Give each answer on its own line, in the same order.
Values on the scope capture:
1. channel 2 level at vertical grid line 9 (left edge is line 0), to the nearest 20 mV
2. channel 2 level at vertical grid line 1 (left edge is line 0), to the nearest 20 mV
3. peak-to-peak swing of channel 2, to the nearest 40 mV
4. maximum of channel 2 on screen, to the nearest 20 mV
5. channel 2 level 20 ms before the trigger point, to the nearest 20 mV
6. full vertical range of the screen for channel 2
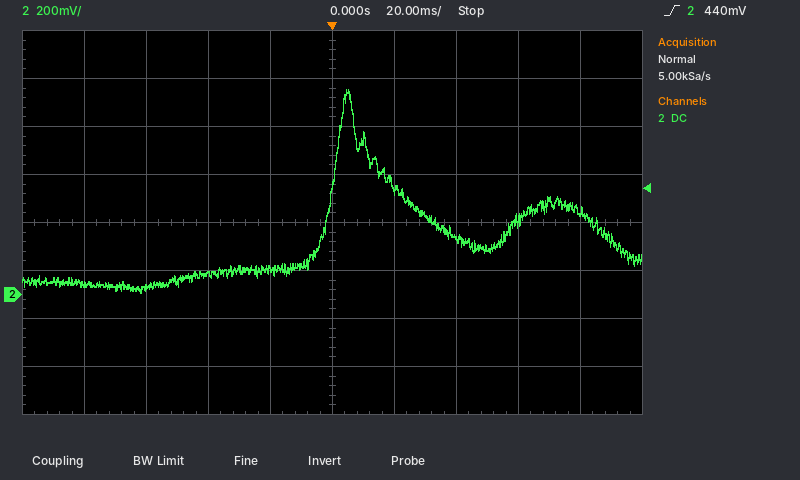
340 mV
40 mV
840 mV
860 mV
100 mV
1.6 V
